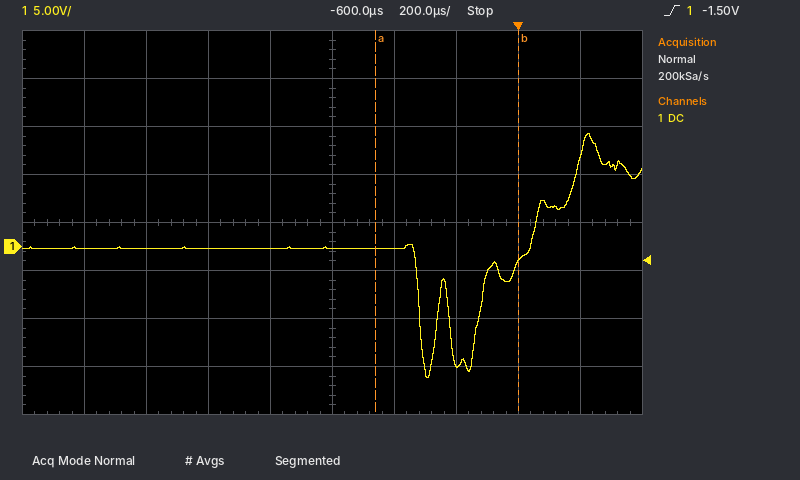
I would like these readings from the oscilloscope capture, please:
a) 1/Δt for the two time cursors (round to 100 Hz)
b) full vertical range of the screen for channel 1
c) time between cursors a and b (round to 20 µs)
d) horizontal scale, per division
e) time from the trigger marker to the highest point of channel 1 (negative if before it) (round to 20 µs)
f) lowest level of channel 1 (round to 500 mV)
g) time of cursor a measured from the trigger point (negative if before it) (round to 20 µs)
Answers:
2.2 kHz
40 V
460 µs
200 µs
+220 µs
-13.5 V
-460 µs
